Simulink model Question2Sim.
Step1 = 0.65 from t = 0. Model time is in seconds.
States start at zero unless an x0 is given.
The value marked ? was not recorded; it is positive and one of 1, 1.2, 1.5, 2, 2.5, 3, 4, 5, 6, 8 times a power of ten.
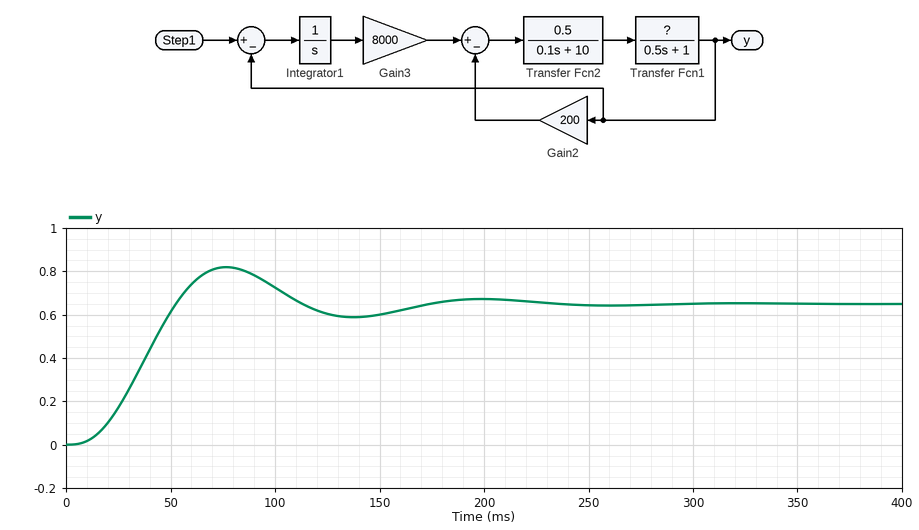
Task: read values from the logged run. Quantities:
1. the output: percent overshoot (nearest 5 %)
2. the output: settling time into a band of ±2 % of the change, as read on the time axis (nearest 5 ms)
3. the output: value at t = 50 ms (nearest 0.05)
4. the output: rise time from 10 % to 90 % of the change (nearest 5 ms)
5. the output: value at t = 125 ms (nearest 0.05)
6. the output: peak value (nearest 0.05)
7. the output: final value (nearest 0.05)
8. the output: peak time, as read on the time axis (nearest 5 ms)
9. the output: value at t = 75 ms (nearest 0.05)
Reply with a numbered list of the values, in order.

1. 25 %
2. 220 ms
3. 0.60
4. 30 ms
5. 0.60
6. 0.80
7. 0.65
8. 75 ms
9. 0.80
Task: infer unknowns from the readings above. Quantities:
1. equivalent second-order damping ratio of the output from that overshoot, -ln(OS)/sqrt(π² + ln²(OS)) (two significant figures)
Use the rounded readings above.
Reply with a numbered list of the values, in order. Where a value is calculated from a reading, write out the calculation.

1. ln(0.25) = -1.386; 1.386 / sqrt(9.870 + 1.922) = 0.40
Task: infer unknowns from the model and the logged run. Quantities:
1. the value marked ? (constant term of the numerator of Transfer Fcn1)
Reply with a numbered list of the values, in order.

1. 2.5
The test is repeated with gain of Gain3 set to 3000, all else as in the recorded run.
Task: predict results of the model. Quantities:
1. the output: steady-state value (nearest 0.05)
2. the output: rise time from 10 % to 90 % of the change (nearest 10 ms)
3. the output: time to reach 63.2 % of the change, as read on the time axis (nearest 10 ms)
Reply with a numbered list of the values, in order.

1. 0.65
2. 100 ms
3. 70 ms
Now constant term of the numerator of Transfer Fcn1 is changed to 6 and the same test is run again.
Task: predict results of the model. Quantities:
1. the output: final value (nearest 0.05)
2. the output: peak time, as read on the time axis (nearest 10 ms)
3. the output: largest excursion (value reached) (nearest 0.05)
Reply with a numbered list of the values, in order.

1. 0.65
2. 50 ms
3. 0.70
